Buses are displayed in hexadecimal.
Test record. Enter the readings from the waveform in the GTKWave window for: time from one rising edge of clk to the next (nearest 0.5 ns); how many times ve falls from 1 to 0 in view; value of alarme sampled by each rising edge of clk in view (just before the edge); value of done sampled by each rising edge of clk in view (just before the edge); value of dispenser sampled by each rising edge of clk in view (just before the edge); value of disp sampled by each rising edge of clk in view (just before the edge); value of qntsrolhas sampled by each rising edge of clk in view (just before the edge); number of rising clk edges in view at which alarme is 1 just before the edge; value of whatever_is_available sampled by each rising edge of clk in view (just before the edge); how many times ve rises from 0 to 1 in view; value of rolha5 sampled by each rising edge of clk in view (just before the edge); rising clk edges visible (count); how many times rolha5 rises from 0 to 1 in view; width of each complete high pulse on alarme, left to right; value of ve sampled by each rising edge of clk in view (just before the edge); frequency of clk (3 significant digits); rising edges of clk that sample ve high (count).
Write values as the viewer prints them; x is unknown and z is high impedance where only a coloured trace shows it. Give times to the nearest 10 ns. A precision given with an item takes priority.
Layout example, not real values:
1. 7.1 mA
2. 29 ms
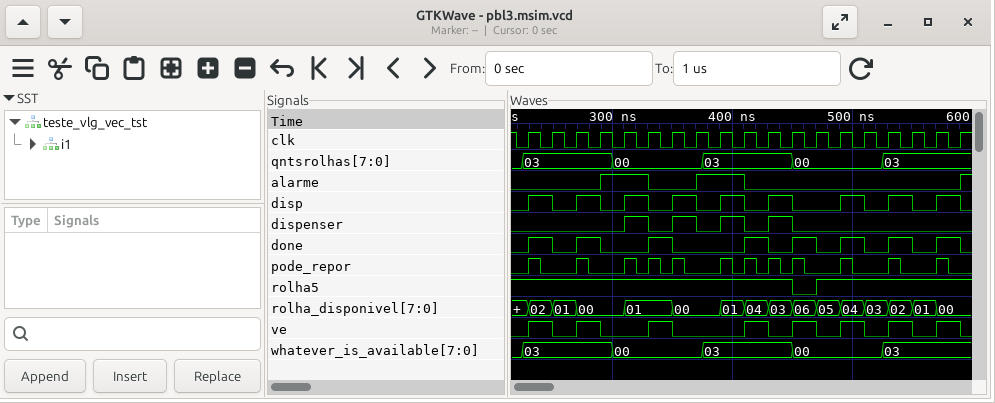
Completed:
1. 20 ns
2. 8
3. 0 0 0 0 1 1 0 0 1 1 0 0 0 0 0 0 0 0 0
4. 0 1 0 1 0 0 1 0 0 0 1 0 1 0 1 0 1 0 1
5. 0 0 0 0 0 1 0 1 0 1 0 1 0 0 0 0 0 0 0
6. 0 1 0 1 0 1 0 1 0 1 0 1 0 0 1 0 1 0 1
7. 03, 03, 03, 03, 00, 00, 00, 00, 03, 03, 03, 03, 00, 00, 00, 03, 03, 03, 03
8. 4
9. 03, 03, 03, 03, 00, 00, 00, 00, 03, 03, 03, 03, 00, 00, 00, 03, 03, 03, 03
10. 8
11. 1 1 1 1 1 1 1 1 1 1 1 1 0 1 1 1 1 1 1
12. 19
13. 1
14. 40 ns, 40 ns
15. 0 1 0 1 0 0 1 0 0 0 1 0 1 0 1 0 1 0 1
16. 50.0 MHz
17. 8
